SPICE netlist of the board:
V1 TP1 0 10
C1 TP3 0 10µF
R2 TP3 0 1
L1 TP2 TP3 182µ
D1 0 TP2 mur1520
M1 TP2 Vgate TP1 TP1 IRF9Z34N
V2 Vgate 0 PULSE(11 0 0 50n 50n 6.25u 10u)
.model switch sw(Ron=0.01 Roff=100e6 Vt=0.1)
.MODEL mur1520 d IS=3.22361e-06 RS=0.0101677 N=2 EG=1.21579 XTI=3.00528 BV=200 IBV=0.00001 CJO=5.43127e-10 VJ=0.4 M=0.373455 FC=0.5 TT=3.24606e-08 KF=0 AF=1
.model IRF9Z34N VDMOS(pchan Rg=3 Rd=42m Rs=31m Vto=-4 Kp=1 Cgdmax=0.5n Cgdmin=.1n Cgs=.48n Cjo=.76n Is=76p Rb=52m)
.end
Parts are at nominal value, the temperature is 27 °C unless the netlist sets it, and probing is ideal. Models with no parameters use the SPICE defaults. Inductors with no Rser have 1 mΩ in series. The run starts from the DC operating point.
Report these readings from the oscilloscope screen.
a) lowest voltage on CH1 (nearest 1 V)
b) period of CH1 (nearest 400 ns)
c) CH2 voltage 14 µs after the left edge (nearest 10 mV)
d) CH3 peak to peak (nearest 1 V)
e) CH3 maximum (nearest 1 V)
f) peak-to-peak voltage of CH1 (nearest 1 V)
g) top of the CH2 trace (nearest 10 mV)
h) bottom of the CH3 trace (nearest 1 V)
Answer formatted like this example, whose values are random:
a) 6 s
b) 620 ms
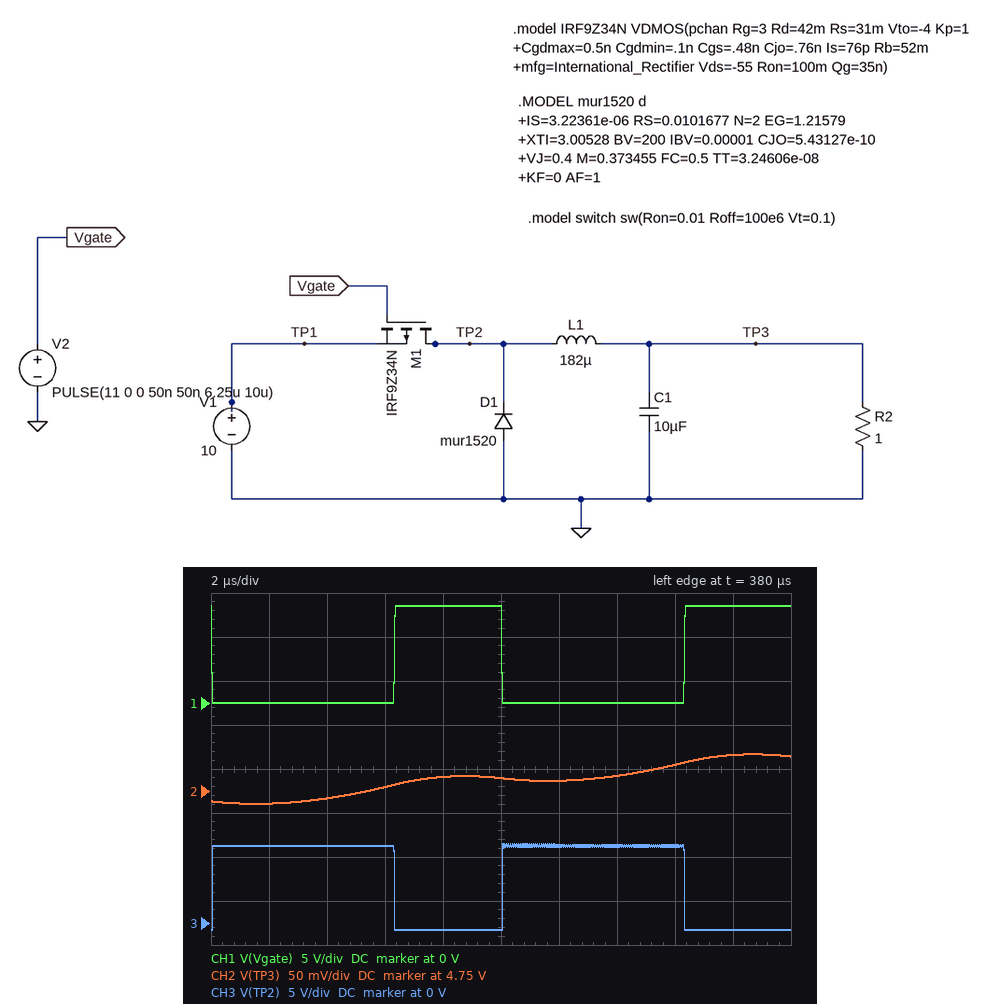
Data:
a) 0 V
b) 10.0 µs
c) 4.77 V
d) 10 V
e) 9 V
f) 11 V
g) 4.79 V
h) -1 V
